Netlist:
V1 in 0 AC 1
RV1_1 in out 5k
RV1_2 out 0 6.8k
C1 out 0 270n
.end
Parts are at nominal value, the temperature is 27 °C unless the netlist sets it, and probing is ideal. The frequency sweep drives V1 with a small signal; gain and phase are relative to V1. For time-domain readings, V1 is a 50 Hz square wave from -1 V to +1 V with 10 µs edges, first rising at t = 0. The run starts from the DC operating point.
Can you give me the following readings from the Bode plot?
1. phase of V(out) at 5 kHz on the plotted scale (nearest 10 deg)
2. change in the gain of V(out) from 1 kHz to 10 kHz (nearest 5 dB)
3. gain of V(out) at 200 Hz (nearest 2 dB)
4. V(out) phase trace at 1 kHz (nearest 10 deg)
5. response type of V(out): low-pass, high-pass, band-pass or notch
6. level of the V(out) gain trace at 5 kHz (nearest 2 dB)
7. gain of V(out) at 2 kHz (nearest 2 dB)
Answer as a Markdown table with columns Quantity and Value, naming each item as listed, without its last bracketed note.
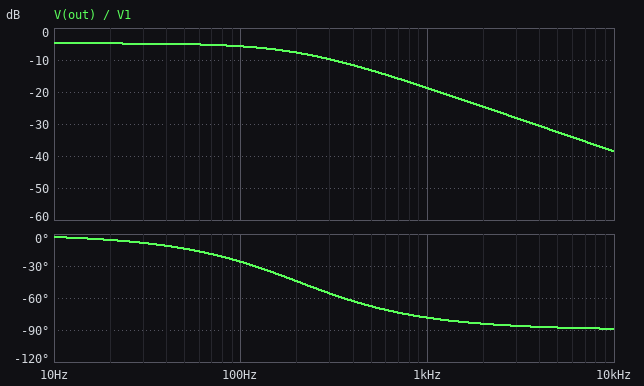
| Quantity | Value |
|---|---|
| phase of V(out) at 5 kHz on the plotted scale | -90 deg |
| change in the gain of V(out) from 1 kHz to 10 kHz | -20 dB |
| gain of V(out) at 200 Hz | -8 dB |
| V(out) phase trace at 1 kHz | -80 deg |
| response type of V(out): low-pass, high-pass, band-pass or notch | low-pass |
| level of the V(out) gain trace at 5 kHz | -32 dB |
| gain of V(out) at 2 kHz | -24 dB |
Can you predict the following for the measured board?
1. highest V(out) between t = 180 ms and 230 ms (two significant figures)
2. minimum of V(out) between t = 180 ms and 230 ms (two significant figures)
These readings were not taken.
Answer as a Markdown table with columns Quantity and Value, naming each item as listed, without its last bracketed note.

| Quantity | Value |
|---|---|
| highest V(out) between t = 180 ms and 230 ms | 580 mV |
| minimum of V(out) between t = 180 ms and 230 ms | -580 mV |
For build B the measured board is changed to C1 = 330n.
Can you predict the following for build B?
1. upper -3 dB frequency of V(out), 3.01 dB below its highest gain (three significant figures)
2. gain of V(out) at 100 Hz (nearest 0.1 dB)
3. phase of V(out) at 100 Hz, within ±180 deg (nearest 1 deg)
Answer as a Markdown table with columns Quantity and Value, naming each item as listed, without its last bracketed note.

| Quantity | Value |
|---|---|
| upper -3 dB frequency of V(out), 3.01 dB below its highest gain | 167 Hz |
| gain of V(out) at 100 Hz | -6.1 dB |
| phase of V(out) at 100 Hz, within ±180 deg | -31 deg |
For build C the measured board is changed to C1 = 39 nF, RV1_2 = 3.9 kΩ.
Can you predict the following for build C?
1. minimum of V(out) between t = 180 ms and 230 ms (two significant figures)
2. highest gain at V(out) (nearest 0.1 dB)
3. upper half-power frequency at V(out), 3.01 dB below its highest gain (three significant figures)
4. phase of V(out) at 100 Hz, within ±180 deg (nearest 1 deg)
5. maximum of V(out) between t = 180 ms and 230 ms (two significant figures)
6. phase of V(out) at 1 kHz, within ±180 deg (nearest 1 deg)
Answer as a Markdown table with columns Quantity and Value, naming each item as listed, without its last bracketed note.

| Quantity | Value |
|---|---|
| minimum of V(out) between t = 180 ms and 230 ms | -440 mV |
| highest gain at V(out) | -7.2 dB |
| upper half-power frequency at V(out), 3.01 dB below its highest gain | 1.86 kHz |
| phase of V(out) at 100 Hz, within ±180 deg | -3 deg |
| maximum of V(out) between t = 180 ms and 230 ms | 440 mV |
| phase of V(out) at 1 kHz, within ±180 deg | -28 deg |
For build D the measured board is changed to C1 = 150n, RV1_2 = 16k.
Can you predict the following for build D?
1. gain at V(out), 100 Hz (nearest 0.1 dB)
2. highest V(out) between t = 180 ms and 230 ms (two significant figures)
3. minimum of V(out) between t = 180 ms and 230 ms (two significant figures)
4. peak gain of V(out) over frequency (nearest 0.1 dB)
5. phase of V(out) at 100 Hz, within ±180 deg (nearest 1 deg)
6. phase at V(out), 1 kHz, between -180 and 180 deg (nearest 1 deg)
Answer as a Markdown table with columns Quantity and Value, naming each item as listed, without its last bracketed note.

| Quantity | Value |
|---|---|
| gain at V(out), 100 Hz | -2.9 dB |
| highest V(out) between t = 180 ms and 230 ms | 760 mV |
| minimum of V(out) between t = 180 ms and 230 ms | -760 mV |
| peak gain of V(out) over frequency | -2.4 dB |
| phase of V(out) at 100 Hz, within ±180 deg | -20 deg |
| phase at V(out), 1 kHz, between -180 and 180 deg | -74 deg |
